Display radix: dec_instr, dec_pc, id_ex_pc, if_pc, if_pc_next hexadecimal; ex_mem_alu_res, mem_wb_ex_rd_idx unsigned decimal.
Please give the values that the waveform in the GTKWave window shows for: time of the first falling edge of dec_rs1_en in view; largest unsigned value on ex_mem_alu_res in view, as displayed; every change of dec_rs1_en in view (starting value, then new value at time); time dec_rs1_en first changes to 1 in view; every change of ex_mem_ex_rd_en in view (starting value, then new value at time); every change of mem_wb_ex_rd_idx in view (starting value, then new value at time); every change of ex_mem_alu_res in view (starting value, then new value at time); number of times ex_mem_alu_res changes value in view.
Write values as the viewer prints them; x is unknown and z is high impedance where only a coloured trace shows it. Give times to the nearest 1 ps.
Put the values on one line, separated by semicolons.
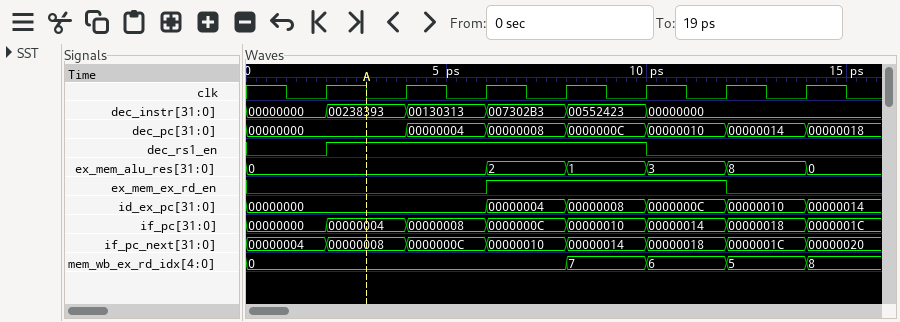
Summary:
10 ps; 8; 0, 1 at 2 ps, 0 at 10 ps; 2 ps; 0, 1 at 6 ps, 0 at 12 ps; 0, 7 at 8 ps, 6 at 10 ps, 5 at 12 ps, 8 at 14 ps; 0, 2 at 6 ps, 1 at 8 ps, 3 at 10 ps, 8 at 12 ps, 0 at 14 ps; 5
